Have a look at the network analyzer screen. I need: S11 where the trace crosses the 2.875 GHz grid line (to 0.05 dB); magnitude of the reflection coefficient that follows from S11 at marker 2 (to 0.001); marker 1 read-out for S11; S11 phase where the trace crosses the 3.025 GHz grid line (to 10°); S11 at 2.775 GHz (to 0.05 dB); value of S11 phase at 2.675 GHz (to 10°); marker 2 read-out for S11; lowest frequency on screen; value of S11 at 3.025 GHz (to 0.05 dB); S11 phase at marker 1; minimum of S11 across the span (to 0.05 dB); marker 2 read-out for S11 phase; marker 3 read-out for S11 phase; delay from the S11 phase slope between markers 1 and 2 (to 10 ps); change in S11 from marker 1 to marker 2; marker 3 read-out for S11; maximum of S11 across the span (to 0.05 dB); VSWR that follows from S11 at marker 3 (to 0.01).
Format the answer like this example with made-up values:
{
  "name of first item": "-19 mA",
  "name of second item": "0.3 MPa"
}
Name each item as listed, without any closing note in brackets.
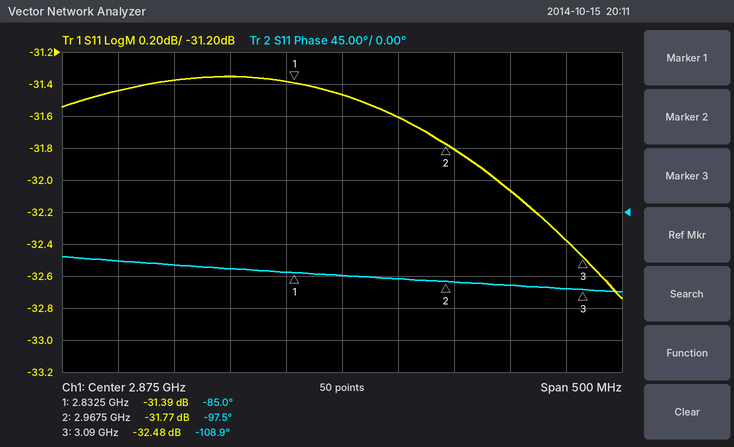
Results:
{
  "S11 where the trace crosses the 2.875 GHz grid line": "-31.45 dB",
  "magnitude of the reflection coefficient that follows from S11 at marker 2": "0.026",
  "marker 1 read-out for S11": "-31.39 dB",
  "S11 phase where the trace crosses the 3.025 GHz grid line": "-100°",
  "S11 at 2.775 GHz": "-31.35 dB",
  "value of S11 phase at 2.675 GHz": "-70°",
  "marker 2 read-out for S11": "-31.77 dB",
  "lowest frequency on screen": "2.625 GHz",
  "value of S11 at 3.025 GHz": "-32.05 dB",
  "S11 phase at marker 1": "-85.0°",
  "minimum of S11 across the span": "-32.75 dB",
  "marker 2 read-out for S11 phase": "-97.5°",
  "marker 3 read-out for S11 phase": "-108.9°",
  "delay from the S11 phase slope between markers 1 and 2": "260 ps",
  "change in S11 from marker 1 to marker 2": "-0.38 dB",
  "marker 3 read-out for S11": "-32.48 dB",
  "maximum of S11 across the span": "-31.35 dB",
  "VSWR that follows from S11 at marker 3": "1.05"
}
